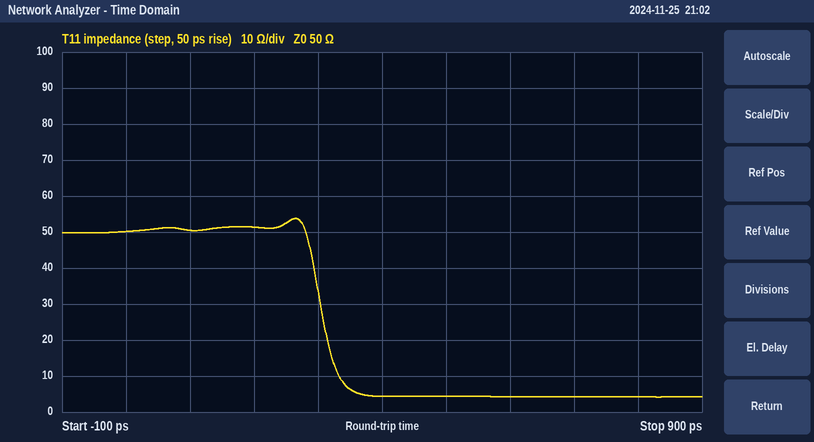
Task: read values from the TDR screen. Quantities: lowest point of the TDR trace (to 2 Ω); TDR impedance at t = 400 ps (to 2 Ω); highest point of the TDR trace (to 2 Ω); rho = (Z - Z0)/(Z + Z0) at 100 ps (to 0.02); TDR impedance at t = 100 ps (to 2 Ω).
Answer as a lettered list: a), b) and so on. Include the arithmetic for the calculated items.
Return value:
a) 4 Ω
b) 4 Ω
c) 54 Ω
d) (50 − 50)/(50 + 50) ≈ 0.00
e) 50 Ω
